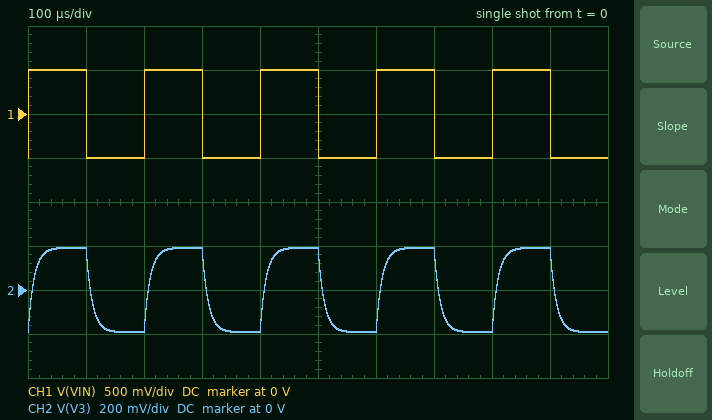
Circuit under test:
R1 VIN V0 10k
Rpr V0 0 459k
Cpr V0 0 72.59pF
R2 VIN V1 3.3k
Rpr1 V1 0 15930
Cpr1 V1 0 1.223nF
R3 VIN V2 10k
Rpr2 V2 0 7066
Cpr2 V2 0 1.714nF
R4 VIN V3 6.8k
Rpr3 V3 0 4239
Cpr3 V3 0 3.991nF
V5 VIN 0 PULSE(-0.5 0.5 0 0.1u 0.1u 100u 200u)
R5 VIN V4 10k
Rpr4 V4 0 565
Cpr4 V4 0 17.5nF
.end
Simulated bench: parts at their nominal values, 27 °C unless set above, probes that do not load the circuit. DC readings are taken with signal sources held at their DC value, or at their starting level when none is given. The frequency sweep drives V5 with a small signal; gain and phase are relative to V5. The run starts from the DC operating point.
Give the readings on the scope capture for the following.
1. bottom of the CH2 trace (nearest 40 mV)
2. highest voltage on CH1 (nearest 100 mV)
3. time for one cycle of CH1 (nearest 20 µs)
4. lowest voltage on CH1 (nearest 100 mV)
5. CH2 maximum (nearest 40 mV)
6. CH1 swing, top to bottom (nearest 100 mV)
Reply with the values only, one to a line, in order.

-200 mV
500 mV
200 µs
-500 mV
200 mV
1.0 V
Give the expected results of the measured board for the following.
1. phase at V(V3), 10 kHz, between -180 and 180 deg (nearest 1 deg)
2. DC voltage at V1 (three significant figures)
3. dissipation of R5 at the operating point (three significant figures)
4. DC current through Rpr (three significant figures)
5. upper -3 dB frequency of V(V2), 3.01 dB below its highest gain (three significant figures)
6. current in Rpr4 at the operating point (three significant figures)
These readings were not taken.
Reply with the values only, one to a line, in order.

-33 deg
-414 mV
22.4 µW
1.07 µA
22.4 kHz
47.3 µA
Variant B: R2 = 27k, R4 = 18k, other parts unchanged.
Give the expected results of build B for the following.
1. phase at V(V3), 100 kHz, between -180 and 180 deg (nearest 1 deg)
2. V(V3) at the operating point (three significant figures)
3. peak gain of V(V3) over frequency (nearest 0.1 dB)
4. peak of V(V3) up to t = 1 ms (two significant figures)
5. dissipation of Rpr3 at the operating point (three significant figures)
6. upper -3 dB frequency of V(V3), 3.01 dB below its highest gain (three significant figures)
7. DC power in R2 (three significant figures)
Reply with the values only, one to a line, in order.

-83 deg
-95.3 mV
-14.4 dB
95 mV
2.14 µW
11.6 kHz
3.66 µW
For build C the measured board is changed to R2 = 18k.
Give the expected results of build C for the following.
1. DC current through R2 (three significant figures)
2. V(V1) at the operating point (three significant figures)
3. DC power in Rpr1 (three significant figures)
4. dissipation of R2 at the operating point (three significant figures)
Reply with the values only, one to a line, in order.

14.7 µA
-235 mV
3.46 µW
3.91 µW
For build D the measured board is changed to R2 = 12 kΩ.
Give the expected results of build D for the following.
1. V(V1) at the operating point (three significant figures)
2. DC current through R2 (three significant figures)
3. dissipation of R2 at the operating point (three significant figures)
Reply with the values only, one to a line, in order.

-285 mV
17.9 µA
3.85 µW
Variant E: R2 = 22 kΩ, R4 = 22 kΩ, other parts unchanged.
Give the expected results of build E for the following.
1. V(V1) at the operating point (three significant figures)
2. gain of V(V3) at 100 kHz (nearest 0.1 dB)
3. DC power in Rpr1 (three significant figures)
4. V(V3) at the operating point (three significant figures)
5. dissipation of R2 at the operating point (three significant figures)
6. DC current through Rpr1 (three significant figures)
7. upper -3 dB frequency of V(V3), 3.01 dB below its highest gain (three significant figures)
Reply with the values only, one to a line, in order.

-210 mV
-34.9 dB
2.77 µW
-80.8 mV
3.82 µW
13.2 µA
11.2 kHz
